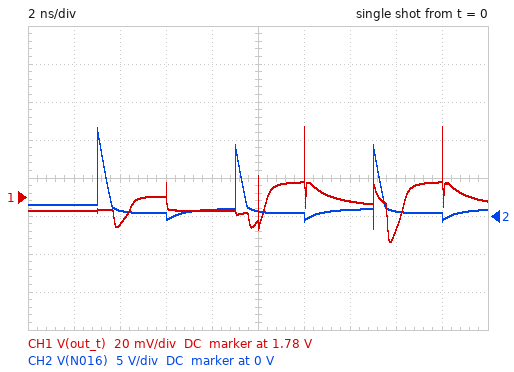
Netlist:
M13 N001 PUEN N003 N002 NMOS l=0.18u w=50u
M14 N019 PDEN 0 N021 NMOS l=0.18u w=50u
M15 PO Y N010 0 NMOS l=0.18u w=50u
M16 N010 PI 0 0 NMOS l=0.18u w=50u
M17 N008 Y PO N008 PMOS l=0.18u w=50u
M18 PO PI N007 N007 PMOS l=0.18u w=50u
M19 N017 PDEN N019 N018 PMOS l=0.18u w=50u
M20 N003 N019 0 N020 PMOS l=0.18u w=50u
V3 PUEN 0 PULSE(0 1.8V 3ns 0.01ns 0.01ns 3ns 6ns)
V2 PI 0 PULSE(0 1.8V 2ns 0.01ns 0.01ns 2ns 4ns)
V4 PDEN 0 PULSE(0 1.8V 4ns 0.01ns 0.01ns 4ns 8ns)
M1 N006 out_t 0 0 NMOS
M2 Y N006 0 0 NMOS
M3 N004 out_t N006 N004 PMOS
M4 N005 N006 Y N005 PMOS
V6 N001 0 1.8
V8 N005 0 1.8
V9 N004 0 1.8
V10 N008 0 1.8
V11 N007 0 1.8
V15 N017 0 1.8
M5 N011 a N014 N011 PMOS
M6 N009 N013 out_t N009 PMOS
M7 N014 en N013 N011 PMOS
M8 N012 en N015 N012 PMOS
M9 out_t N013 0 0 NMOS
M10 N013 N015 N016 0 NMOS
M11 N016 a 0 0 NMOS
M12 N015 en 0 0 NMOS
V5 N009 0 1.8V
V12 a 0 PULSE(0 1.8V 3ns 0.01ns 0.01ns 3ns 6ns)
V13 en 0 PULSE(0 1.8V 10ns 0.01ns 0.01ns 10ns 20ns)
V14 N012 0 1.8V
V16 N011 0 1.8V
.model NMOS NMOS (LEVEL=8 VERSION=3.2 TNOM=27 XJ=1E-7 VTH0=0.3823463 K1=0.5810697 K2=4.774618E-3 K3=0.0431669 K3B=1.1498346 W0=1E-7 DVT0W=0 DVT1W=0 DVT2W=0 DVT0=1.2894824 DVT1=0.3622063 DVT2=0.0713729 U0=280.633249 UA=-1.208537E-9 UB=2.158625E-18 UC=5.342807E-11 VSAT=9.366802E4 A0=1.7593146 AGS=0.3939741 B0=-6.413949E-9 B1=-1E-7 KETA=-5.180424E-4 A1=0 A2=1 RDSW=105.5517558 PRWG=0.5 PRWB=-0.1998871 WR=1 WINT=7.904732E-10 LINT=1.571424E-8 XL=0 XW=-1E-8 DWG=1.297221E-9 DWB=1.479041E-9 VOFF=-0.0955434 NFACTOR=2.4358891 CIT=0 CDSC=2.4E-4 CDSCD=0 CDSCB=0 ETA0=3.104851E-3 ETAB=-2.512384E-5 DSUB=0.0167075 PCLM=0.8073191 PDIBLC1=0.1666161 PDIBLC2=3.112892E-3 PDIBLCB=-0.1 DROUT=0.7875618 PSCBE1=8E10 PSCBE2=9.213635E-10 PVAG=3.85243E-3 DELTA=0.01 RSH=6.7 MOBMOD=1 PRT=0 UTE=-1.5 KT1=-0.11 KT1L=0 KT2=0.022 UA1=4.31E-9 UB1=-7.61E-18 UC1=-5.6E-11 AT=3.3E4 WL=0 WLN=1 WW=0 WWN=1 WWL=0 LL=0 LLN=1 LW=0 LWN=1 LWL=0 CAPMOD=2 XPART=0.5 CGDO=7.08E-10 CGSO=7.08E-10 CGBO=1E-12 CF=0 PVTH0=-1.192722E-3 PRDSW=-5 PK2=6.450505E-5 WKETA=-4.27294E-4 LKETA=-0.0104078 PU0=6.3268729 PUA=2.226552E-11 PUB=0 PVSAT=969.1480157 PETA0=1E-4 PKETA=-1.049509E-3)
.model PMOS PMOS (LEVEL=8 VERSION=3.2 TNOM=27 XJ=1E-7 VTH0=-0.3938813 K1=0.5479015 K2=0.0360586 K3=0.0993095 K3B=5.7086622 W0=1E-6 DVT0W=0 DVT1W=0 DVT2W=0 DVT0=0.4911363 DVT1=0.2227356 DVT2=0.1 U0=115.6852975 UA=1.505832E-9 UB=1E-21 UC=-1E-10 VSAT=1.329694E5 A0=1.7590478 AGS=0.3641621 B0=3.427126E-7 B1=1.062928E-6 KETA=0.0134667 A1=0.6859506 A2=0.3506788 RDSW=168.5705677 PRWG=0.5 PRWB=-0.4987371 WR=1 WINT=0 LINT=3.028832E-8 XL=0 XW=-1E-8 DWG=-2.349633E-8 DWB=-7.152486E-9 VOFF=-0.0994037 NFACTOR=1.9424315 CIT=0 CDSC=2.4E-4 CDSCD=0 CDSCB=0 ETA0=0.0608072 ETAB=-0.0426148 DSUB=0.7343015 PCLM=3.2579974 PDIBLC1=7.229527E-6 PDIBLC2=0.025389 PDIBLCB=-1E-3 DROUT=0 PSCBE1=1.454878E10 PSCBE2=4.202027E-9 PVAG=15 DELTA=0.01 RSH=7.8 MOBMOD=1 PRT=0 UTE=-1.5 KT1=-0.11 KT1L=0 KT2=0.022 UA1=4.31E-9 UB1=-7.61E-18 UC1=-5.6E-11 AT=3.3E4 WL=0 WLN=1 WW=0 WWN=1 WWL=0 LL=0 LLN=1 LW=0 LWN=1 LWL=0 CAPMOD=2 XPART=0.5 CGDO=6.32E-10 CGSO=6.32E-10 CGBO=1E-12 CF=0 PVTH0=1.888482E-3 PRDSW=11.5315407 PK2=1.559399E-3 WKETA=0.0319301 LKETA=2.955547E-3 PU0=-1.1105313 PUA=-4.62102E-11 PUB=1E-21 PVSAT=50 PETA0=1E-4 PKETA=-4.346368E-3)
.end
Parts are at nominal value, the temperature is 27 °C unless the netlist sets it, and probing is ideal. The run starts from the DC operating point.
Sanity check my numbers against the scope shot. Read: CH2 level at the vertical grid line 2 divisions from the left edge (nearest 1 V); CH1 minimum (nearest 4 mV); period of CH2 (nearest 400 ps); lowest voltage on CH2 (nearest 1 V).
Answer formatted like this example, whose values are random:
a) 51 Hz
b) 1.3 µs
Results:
a) 1 V
b) 1.756 V
c) 6.0 ns
d) -1 V
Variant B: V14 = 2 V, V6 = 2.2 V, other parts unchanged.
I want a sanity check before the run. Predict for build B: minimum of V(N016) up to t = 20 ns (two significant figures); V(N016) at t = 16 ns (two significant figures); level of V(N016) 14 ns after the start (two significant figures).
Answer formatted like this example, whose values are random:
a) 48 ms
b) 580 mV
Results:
a) -470 mV
b) 700 mV
c) 970 mV
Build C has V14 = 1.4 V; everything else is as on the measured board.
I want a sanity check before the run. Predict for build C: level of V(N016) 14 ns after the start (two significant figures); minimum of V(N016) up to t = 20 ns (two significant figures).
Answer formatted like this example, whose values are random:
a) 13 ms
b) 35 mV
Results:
a) -480 mV
b) -1.3 V
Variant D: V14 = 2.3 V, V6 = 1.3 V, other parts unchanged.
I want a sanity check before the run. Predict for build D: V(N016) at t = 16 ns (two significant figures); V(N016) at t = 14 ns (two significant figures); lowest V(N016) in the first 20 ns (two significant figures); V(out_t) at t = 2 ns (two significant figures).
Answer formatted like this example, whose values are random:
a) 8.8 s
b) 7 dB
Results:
a) 880 mV
b) 1.2 V
c) -380 mV
d) 1.8 V
